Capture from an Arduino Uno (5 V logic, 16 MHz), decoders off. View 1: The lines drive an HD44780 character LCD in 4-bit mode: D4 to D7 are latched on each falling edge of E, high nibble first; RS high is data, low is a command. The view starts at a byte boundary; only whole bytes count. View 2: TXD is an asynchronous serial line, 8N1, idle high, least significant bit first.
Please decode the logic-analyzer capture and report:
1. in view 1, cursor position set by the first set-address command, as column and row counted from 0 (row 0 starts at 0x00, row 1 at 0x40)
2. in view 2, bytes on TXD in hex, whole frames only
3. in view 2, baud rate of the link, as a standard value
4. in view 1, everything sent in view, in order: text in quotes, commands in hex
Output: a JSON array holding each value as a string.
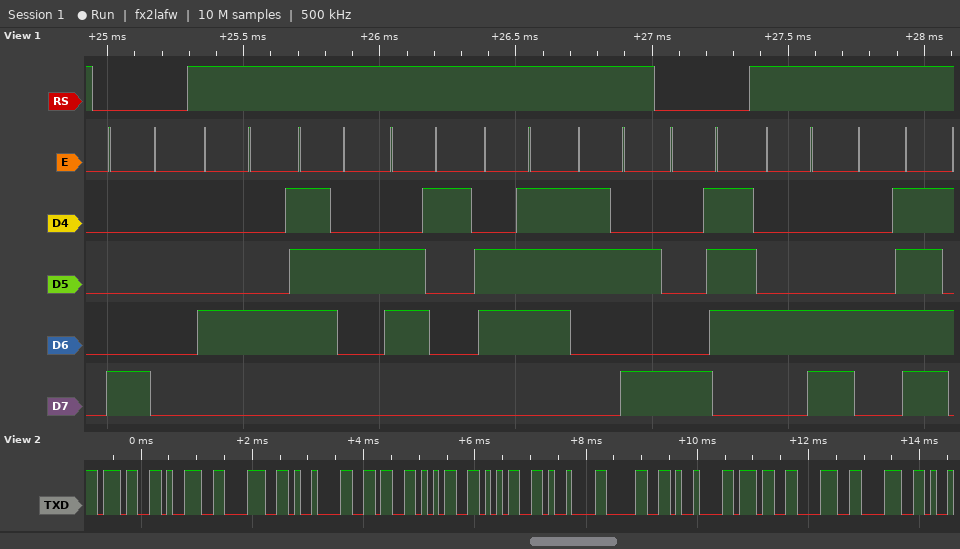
["column 0, row 0", "0x37 0x39 0x38 0x09 0x36 0x35 0x35 0x09 0x30 0x09 0x37 0x38 0x38", "9600 baud", "0x80 \"Drag:\" 0x87 \"LO\""]
